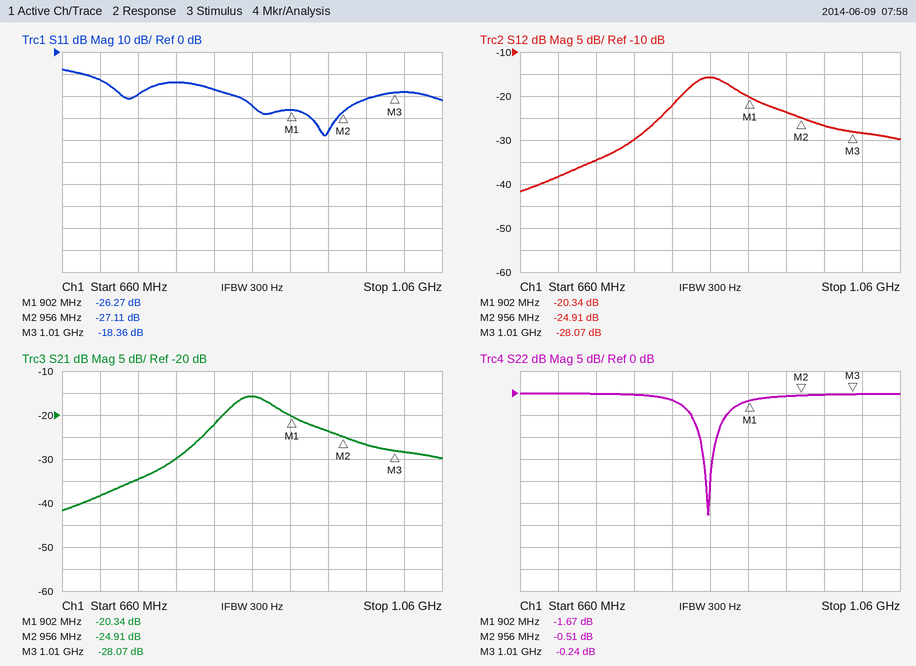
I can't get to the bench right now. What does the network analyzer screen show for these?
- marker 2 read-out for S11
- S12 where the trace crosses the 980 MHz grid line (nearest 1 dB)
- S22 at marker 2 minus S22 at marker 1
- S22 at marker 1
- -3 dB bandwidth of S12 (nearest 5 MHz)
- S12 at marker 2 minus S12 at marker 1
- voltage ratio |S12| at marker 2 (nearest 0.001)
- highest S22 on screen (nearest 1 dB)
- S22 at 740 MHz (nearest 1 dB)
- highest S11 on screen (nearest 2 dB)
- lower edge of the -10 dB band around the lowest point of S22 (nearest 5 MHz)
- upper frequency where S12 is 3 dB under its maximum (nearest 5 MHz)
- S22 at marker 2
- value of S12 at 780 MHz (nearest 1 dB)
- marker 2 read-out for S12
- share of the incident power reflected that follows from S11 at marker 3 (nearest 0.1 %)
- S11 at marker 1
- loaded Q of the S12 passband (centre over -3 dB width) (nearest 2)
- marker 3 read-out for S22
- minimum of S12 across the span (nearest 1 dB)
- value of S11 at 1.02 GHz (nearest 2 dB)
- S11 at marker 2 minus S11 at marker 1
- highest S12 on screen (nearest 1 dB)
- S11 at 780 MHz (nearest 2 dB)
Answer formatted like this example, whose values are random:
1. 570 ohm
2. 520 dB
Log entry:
1. -27.11 dB
2. -27 dB
3. 1.16 dB
4. -1.67 dB
5. 55 MHz
6. -4.57 dB
7. 0.057
8. 0 dB
9. 0 dB
10. -8 dB
11. 850 MHz
12. 890 MHz
13. -0.51 dB
14. -30 dB
15. -24.91 dB
16. 1.5 %
17. -26.27 dB
18. 16
19. -0.24 dB
20. -42 dB
21. -18 dB
22. -0.84 dB
23. -16 dB
24. -14 dB
